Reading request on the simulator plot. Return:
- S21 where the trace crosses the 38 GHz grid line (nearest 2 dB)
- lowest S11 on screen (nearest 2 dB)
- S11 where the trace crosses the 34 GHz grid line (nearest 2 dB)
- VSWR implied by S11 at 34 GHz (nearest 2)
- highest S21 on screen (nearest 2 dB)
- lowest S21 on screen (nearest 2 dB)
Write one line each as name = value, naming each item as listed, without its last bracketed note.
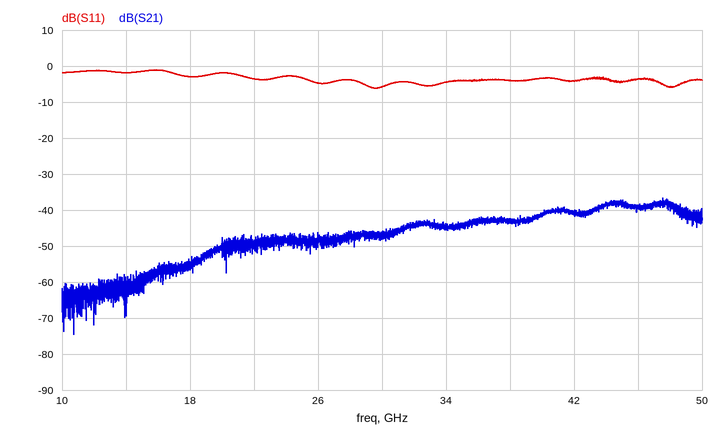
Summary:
S21 where the trace crosses the 38 GHz grid line = -42 dB
lowest S11 on screen = -6 dB
S11 where the trace crosses the 34 GHz grid line = -4 dB
VSWR implied by S11 at 34 GHz = 4
highest S21 on screen = -36 dB
lowest S21 on screen = -74 dB
